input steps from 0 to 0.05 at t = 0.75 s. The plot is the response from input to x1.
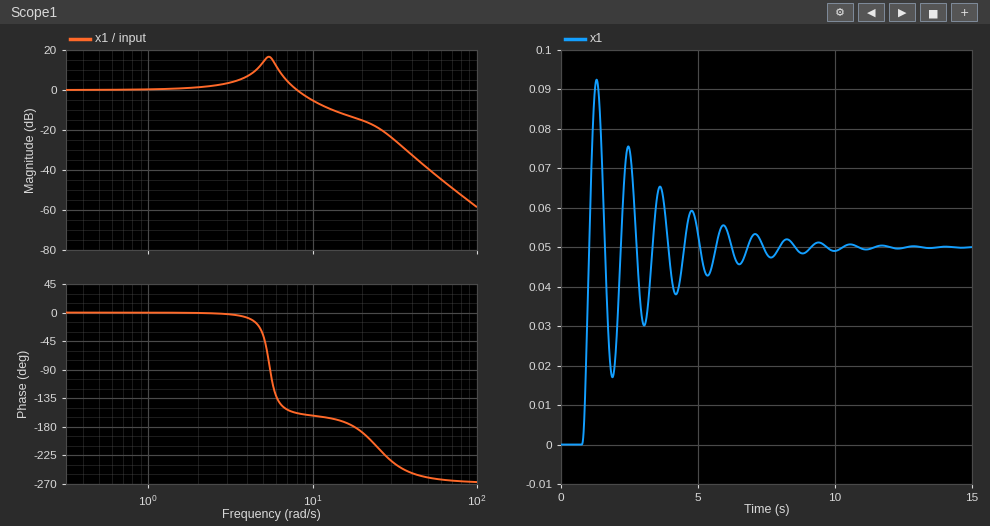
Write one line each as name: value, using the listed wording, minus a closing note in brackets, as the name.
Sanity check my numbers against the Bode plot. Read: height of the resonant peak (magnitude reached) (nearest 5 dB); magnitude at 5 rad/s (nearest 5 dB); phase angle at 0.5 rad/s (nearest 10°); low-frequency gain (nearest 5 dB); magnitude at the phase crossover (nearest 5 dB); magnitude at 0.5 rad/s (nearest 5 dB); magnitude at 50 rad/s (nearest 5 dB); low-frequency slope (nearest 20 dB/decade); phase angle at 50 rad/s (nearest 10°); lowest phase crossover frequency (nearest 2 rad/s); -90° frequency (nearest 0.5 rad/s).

height of the resonant peak (magnitude reached): 15 dB
magnitude at 5 rad/s: 15 dB
phase angle at 0.5 rad/s: 0°
low-frequency gain: 0 dB
magnitude at the phase crossover: -15 dB
magnitude at 0.5 rad/s: 0 dB
magnitude at 50 rad/s: -40 dB
low-frequency slope: 0 dB/decade
phase angle at 50 rad/s: -260°
lowest phase crossover frequency: 18 rad/s
-90° frequency: 5.5 rad/s
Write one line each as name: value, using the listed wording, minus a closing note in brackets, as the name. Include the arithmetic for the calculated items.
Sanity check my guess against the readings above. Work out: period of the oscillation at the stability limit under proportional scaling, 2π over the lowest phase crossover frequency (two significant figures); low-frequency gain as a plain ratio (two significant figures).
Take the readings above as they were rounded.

period of the oscillation at the stability limit under proportional scaling, 2π over the lowest phase crossover frequency: 2π / 18 = 0.35 s
low-frequency gain as a plain ratio: 10^(0 / 20) = 1.0
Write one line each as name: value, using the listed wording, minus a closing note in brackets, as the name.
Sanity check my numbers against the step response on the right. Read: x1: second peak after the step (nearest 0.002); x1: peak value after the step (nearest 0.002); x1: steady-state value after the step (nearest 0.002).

x1: second peak after the step: 0.076
x1: peak value after the step: 0.092
x1: steady-state value after the step: 0.050
